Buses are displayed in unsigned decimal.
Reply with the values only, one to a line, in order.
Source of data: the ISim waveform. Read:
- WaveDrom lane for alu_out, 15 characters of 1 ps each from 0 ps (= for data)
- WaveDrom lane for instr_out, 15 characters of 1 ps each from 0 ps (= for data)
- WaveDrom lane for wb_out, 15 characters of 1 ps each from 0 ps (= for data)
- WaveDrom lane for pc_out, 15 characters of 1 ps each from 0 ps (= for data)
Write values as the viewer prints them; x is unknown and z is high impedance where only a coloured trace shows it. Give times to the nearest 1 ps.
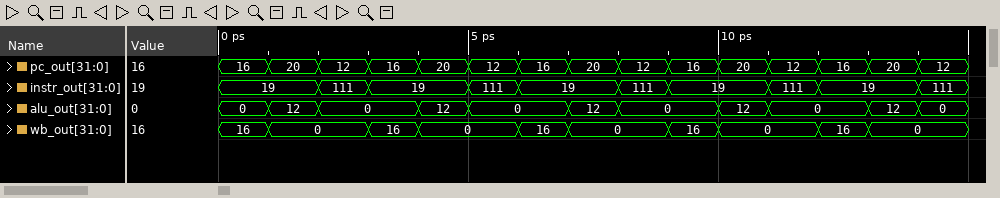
{name: 'alu_out', wave: '===.==.==.==.==', data: '0 12 0 12 0 12 0 12 0 12 0'}
{name: 'instr_out', wave: '=.==.==.==.==.=', data: '19 111 19 111 19 111 19 111 19 111'}
{name: 'wb_out', wave: '==.==.==.==.==.', data: '16 0 16 0 16 0 16 0 16 0'}
{name: 'pc_out', wave: '===============', data: '16 20 12 16 20 12 16 20 12 16 20 12 16 20 12'}
